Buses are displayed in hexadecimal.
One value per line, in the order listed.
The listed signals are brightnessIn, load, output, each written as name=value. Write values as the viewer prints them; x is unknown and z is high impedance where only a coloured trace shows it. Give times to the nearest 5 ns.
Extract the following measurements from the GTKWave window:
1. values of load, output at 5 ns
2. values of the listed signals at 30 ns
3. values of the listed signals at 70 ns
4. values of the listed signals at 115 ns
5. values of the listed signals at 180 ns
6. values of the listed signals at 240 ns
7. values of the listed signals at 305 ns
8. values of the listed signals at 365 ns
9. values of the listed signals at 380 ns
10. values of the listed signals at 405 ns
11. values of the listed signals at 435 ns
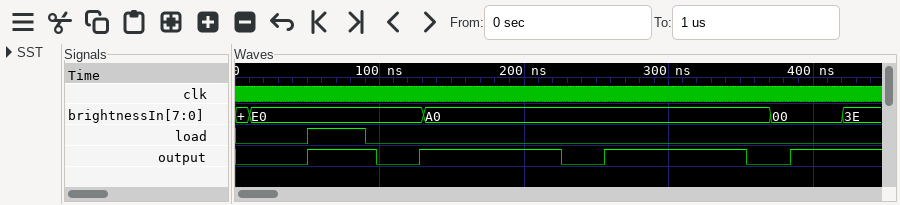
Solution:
load=0, output=0
brightnessIn=E0, load=0, output=0
brightnessIn=E0, load=1, output=1
brightnessIn=E0, load=0, output=0
brightnessIn=A0, load=0, output=1
brightnessIn=A0, load=0, output=0
brightnessIn=A0, load=0, output=1
brightnessIn=A0, load=0, output=0
brightnessIn=00, load=0, output=0
brightnessIn=00, load=0, output=1
brightnessIn=3E, load=0, output=1
